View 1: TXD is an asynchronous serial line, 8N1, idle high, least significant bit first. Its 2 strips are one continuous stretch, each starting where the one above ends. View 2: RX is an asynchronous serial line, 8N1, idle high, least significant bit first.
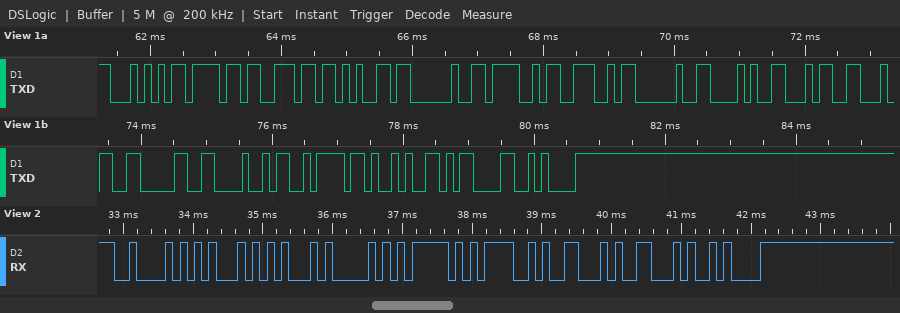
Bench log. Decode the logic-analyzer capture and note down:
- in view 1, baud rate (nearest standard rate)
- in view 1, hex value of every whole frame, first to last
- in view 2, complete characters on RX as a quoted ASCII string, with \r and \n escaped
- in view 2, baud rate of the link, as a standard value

9600 baud
54 6F 6E 65 20 4F 4E 20 28 34 34 30 48 7A 29 0D 0A
"BEEP_OFF\n"
9600 baud
